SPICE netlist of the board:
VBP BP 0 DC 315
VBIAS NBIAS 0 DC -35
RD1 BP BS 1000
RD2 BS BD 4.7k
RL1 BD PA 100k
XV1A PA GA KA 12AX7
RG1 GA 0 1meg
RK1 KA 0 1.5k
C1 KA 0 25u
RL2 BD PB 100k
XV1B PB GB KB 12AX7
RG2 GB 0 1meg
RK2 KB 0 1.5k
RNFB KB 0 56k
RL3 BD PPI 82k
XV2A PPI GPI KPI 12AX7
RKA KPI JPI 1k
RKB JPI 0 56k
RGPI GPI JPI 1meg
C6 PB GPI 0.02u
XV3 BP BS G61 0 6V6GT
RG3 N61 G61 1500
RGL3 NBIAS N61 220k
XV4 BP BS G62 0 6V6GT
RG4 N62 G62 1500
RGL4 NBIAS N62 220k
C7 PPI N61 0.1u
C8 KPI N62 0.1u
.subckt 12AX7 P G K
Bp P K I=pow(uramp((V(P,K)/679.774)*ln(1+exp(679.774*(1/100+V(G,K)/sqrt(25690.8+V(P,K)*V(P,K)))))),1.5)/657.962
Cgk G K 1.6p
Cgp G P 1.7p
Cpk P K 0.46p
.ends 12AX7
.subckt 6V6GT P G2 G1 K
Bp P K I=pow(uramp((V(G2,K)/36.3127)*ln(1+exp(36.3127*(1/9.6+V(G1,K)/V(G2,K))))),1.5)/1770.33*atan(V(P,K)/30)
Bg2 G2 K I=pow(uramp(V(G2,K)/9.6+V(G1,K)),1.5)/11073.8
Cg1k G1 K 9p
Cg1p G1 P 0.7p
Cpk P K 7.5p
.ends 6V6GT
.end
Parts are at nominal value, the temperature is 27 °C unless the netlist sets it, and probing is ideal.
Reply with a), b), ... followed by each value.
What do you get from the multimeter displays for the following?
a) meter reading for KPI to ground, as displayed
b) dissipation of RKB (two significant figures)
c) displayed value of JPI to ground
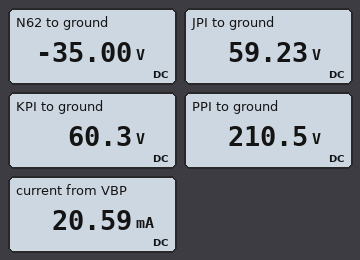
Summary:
a) 60.3 V
b) 63 mW
c) 59.23 V
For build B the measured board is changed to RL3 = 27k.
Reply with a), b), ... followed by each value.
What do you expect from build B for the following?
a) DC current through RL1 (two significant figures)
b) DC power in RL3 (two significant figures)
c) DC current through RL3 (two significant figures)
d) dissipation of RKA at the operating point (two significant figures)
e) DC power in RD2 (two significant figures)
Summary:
a) 1.0 mA
b) 45 mW
c) 1.3 mA
d) 1.7 mW
e) 53 mW
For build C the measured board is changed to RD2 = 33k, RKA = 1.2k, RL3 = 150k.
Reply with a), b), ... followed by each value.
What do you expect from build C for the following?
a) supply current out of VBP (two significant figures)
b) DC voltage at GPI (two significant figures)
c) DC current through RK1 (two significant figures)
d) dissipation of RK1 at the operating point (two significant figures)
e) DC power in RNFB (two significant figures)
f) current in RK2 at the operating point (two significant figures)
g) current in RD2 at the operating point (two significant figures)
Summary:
a) 20 mA
b) 37 V
c) 830 µA
d) 1.0 mW
e) 27 µW
f) 820 µA
g) 2.3 mA
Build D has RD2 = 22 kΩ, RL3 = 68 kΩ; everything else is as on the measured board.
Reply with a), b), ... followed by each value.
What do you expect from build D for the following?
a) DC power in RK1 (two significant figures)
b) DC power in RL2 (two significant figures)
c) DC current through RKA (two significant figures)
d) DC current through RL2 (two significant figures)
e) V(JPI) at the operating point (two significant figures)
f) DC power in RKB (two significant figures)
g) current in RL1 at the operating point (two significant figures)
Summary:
a) 1.2 mW
b) 80 mW
c) 950 µA
d) 890 µA
e) 53 V
f) 51 mW
g) 880 µA
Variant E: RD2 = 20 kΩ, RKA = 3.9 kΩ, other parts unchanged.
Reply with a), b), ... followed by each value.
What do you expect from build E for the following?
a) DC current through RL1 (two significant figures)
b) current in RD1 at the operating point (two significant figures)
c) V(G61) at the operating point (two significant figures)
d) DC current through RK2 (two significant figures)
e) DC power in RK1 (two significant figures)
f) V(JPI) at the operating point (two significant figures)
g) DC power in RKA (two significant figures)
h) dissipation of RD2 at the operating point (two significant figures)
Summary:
a) 920 µA
b) 2.4 mA
c) -35 V
d) 910 µA
e) 1.3 mW
f) 28 V
g) 990 µW
h) 110 mW
